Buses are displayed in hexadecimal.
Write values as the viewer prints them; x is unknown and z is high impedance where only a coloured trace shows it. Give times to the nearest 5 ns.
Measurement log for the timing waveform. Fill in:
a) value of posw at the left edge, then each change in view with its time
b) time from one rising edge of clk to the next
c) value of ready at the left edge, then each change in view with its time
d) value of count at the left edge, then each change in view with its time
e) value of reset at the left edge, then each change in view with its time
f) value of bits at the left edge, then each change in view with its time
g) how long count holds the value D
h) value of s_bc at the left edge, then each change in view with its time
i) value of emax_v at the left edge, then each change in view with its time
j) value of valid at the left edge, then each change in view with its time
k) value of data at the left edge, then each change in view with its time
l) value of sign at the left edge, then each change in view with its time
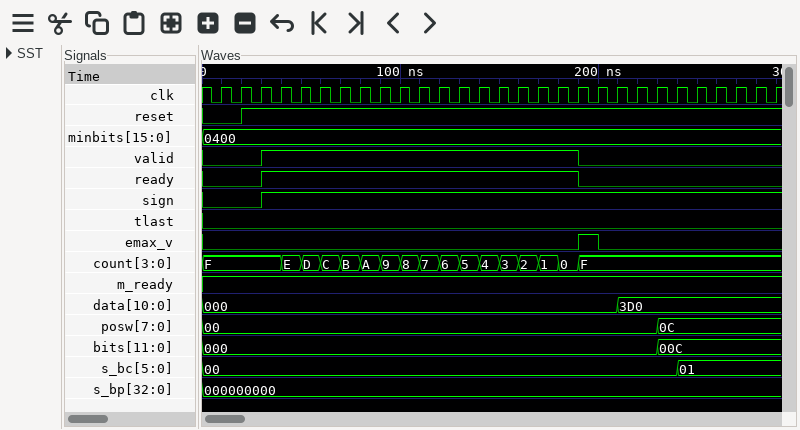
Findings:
00, 0C at 230 ns
10 ns
0, 1 at 30 ns, 0 at 190 ns
F, E at 40 ns, D at 50 ns, C at 60 ns, B at 70 ns, A at 80 ns, 9 at 90 ns, 8 at 100 ns, 7 at 110 ns, 6 at 120 ns, 5 at 130 ns, 4 at 140 ns, 3 at 150 ns, 2 at 160 ns, 1 at 170 ns, 0 at 180 ns, F at 190 ns
0, 1 at 20 ns
000, 00C at 230 ns
10 ns
00, 01 at 240 ns
0, 1 at 190 ns, 0 at 200 ns
0, 1 at 30 ns, 0 at 190 ns
000, 3D0 at 210 ns
0, 1 at 30 ns
